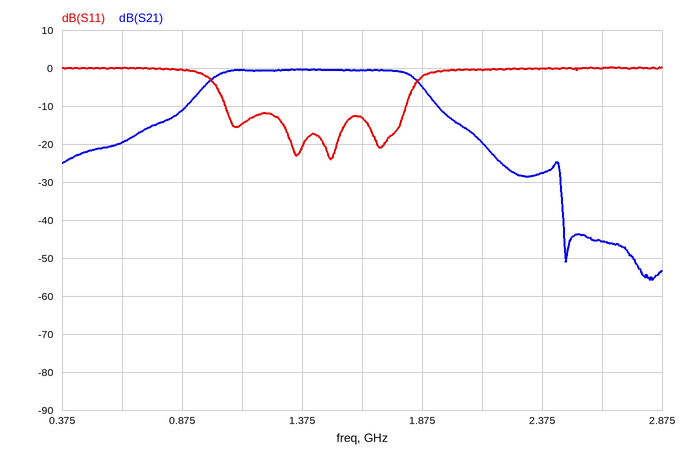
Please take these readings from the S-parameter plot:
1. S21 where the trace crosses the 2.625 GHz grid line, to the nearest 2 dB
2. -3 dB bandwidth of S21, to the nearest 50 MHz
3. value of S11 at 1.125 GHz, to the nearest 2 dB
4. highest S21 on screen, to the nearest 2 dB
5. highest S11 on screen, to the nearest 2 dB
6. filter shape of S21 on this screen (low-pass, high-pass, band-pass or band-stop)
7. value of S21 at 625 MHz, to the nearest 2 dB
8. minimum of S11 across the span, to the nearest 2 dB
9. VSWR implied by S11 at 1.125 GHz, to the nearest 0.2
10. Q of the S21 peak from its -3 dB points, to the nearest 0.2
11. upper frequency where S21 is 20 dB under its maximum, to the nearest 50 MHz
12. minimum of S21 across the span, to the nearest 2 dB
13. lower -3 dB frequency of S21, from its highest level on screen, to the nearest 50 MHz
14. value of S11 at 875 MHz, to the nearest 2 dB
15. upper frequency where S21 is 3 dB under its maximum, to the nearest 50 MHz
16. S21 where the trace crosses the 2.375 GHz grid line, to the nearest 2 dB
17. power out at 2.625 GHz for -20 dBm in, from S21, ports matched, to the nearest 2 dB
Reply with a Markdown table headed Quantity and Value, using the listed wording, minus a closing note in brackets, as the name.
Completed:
| Quantity | Value |
|---|---|
| S21 where the trace crosses the 2.625 GHz grid line, to the nearest 2 dB | -46 dB |
| -3 dB bandwidth of S21, to the nearest 50 MHz | 850 MHz |
| value of S11 at 1.125 GHz, to the nearest 2 dB | -14 dB |
| highest S21 on screen, to the nearest 2 dB | 0 dB |
| highest S11 on screen, to the nearest 2 dB | 0 dB |
| filter shape of S21 on this screen | band-pass |
| value of S21 at 625 MHz, to the nearest 2 dB | -20 dB |
| minimum of S11 across the span, to the nearest 2 dB | -24 dB |
| VSWR implied by S11 at 1.125 GHz, to the nearest 0.2 | 1.4 |
| Q of the S21 peak from its -3 dB points, to the nearest 0.2 | 1.6 |
| upper frequency where S21 is 20 dB under its maximum, to the nearest 50 MHz | 2.15 GHz |
| minimum of S21 across the span, to the nearest 2 dB | -56 dB |
| lower -3 dB frequency of S21, from its highest level on screen, to the nearest 50 MHz | 1.00 GHz |
| value of S11 at 875 MHz, to the nearest 2 dB | 0 dB |
| upper frequency where S21 is 3 dB under its maximum, to the nearest 50 MHz | 1.85 GHz |
| S21 where the trace crosses the 2.375 GHz grid line, to the nearest 2 dB | -28 dB |
| power out at 2.625 GHz for -20 dBm in, from S21, ports matched, to the nearest 2 dB | -66 dBm |
